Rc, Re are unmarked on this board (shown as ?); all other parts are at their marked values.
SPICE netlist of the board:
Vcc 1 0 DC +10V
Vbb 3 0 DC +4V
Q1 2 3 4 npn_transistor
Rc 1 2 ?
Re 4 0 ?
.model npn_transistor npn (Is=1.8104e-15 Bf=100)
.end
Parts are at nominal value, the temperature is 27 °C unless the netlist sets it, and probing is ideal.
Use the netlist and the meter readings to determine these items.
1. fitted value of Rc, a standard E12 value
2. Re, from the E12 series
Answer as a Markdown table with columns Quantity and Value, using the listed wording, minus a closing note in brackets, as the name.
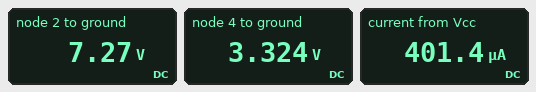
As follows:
| Quantity | Value |
|---|---|
| fitted value of Rc, a standard E12 value | 6.8 kΩ |
| Re, from the E12 series | 8.2 kΩ |
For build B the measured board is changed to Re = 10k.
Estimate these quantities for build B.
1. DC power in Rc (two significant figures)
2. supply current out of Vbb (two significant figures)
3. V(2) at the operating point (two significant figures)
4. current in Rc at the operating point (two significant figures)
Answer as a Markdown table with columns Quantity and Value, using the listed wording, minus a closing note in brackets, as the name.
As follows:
| Quantity | Value |
|---|---|
| DC power in Rc | 740 µW |
| supply current out of Vbb | 3.3 µA |
| V(2) at the operating point | 7.8 V |
| current in Rc at the operating point | 330 µA |
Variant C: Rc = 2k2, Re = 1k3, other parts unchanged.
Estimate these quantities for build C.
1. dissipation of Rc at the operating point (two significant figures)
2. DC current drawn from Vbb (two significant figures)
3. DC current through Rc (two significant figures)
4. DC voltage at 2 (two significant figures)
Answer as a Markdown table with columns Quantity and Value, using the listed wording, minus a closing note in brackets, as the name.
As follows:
| Quantity | Value |
|---|---|
| dissipation of Rc at the operating point | 14 mW |
| DC current drawn from Vbb | 25 µA |
| DC current through Rc | 2.5 mA |
| DC voltage at 2 | 4.5 V |
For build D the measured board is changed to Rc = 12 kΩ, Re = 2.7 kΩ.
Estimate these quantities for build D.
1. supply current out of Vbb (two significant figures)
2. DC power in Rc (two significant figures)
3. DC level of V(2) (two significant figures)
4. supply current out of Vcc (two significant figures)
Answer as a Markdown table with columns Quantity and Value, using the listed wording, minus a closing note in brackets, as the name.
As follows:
| Quantity | Value |
|---|---|
| supply current out of Vbb | 660 µA |
| DC power in Rc | 3.7 mW |
| DC level of V(2) | 3.3 V |
| supply current out of Vcc | 560 µA |
